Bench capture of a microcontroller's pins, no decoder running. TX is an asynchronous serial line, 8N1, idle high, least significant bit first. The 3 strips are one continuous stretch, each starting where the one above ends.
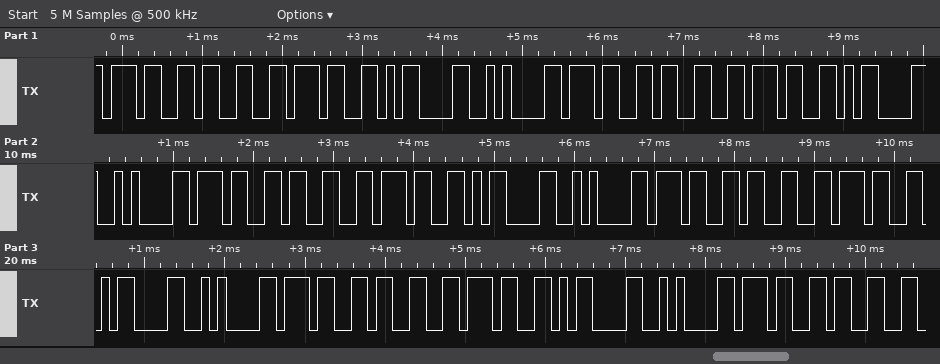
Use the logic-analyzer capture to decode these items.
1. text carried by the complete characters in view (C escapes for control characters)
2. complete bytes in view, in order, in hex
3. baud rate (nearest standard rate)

"737\r\n737\r\n737\r\n737\r\n737\r\n73"
37 33 37 0D 0A 37 33 37 0D 0A 37 33 37 0D 0A 37 33 37 0D 0A 37 33 37 0D 0A 37 33
9600 baud
